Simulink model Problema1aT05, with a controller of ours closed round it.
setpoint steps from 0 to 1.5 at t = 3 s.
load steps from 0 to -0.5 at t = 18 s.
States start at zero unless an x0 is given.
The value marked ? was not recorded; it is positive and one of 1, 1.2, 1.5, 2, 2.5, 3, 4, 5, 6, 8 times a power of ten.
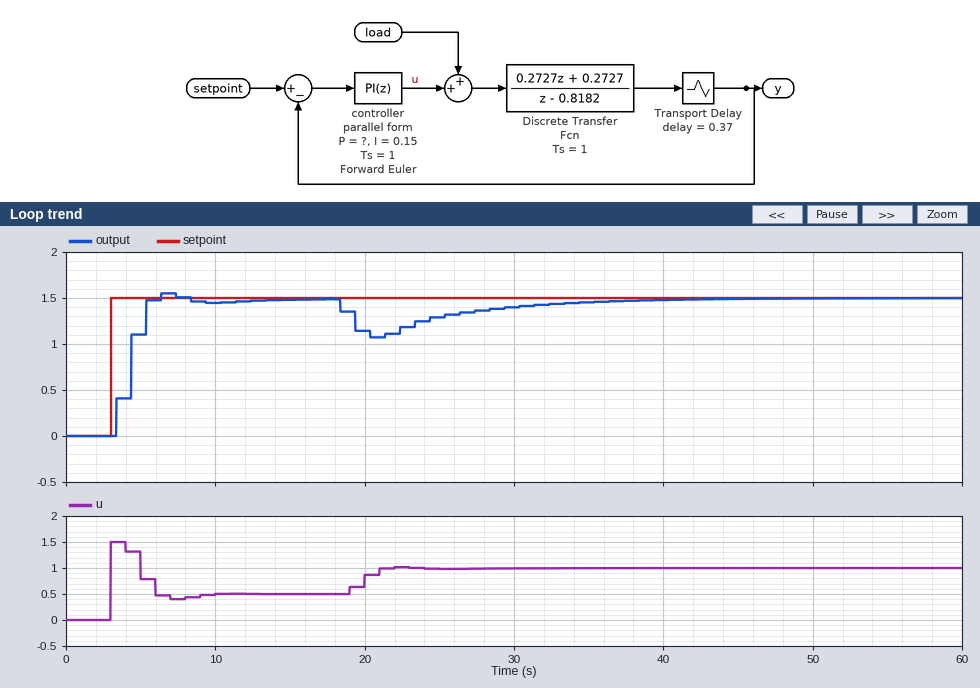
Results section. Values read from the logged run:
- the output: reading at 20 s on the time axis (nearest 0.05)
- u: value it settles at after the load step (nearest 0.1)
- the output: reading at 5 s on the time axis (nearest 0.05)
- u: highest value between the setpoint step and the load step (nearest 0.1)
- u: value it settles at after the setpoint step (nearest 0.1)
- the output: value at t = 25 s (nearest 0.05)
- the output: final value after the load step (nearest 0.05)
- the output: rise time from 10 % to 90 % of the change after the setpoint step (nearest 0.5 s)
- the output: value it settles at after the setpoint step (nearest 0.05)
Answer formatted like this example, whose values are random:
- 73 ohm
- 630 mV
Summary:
- 1.15
- 1.0
- 1.10
- 1.5
- 0.5
- 1.30
- 1.50
- 2.0 s
- 1.50
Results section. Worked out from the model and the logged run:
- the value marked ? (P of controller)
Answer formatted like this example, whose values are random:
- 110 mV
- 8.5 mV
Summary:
- 1
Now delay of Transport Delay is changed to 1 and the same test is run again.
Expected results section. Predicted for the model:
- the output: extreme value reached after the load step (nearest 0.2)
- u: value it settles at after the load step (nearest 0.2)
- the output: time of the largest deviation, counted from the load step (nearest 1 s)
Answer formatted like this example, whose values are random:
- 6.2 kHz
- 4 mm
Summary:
- 1.0
- 1.0
- 3 s
